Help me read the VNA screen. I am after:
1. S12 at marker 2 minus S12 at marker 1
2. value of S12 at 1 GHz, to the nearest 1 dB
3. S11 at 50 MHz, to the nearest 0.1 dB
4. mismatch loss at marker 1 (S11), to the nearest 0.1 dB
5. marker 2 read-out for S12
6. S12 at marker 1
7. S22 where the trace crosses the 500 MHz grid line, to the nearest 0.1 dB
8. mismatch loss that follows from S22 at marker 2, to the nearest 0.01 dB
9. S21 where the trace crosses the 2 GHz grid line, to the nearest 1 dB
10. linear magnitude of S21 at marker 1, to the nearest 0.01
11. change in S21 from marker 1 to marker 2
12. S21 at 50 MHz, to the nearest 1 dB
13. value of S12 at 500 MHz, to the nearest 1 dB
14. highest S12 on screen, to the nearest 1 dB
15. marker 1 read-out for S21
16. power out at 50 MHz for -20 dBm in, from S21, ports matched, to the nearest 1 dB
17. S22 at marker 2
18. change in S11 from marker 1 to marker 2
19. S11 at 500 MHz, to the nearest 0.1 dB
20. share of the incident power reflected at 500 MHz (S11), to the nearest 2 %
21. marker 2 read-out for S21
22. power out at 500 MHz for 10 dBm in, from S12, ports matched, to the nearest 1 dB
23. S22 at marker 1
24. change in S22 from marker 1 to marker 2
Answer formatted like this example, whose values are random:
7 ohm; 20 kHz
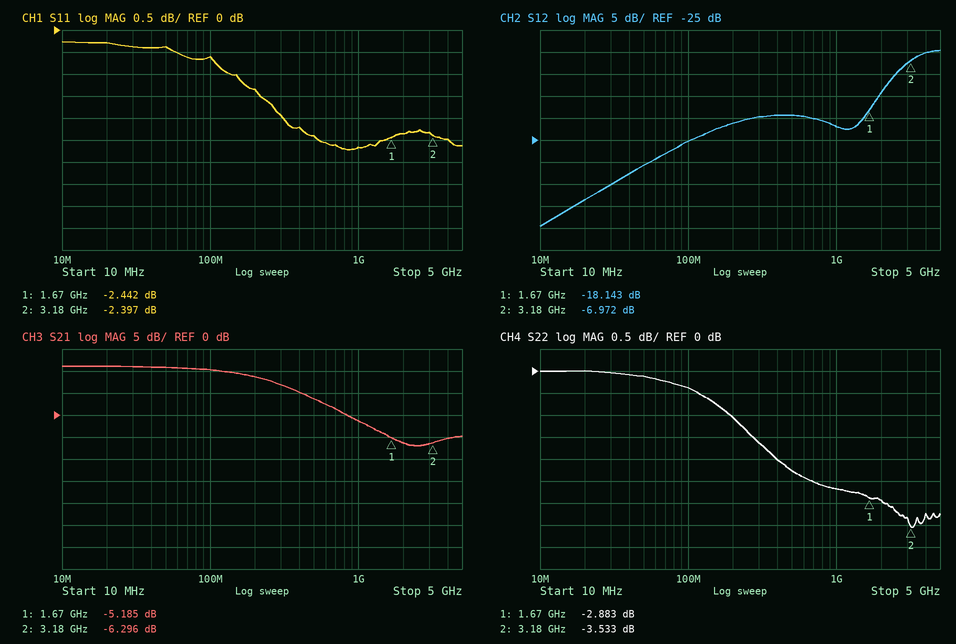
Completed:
11.171 dB; -22 dB; -0.4 dB; 3.7 dB; -6.972 dB; -18.143 dB; -2.3 dB; 2.54 dB; -6 dB; 0.55; -1.111 dB; 11 dB; -19 dB; -5 dB; -5.185 dB; -9 dBm; -3.533 dB; 0.045 dB; -2.4 dB; 58 %; -6.296 dB; -9 dBm; -2.883 dB; -0.650 dB
